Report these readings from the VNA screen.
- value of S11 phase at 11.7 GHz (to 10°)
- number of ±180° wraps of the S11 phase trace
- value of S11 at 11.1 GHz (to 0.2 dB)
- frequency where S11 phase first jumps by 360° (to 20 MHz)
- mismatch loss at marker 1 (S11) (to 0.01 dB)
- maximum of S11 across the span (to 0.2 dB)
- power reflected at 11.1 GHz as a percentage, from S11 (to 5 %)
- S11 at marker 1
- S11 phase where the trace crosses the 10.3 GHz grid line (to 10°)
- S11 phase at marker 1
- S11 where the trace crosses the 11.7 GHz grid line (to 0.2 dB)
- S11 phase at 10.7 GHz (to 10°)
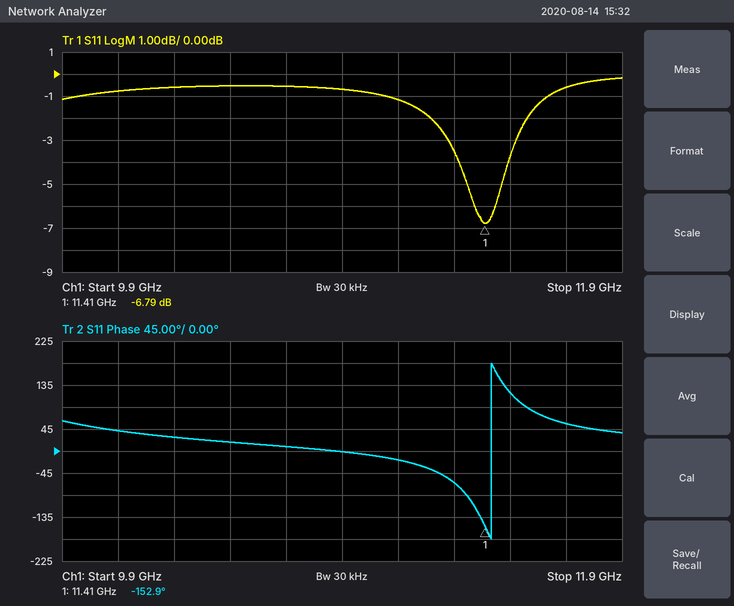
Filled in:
60°
1
-1.2 dB
11.44 GHz
1.02 dB
-0.2 dB
75 %
-6.79 dB
30°
-152.9°
-0.6 dB
10°
